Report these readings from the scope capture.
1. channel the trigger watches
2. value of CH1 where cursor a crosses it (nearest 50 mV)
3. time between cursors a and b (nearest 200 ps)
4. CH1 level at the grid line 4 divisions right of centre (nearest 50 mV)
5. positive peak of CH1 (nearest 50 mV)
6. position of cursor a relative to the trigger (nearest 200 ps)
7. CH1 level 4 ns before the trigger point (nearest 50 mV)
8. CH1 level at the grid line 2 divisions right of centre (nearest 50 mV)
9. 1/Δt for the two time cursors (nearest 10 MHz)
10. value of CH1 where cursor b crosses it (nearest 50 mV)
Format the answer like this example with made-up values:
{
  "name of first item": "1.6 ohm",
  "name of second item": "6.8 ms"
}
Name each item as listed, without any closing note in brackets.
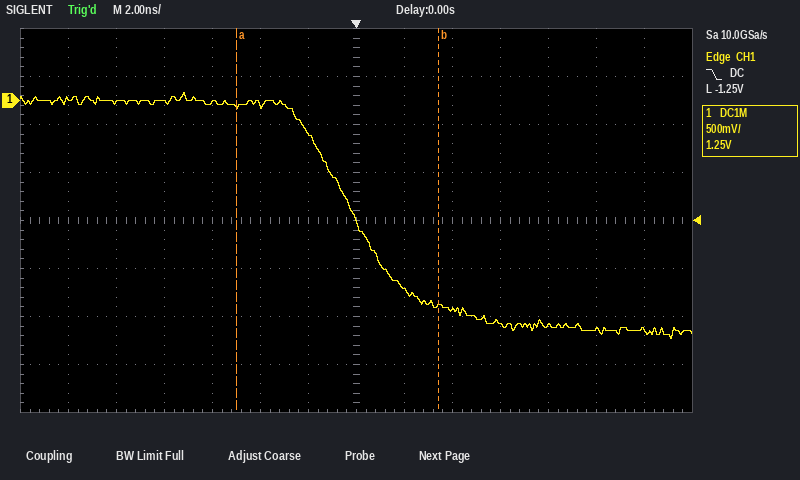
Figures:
{
  "channel the trigger watches": "CH1",
  "value of CH1 where cursor a crosses it": "-50 mV",
  "time between cursors a and b": "8.4 ns",
  "CH1 level at the grid line 4 divisions right of centre": "-2.35 V",
  "positive peak of CH1": "100 mV",
  "position of cursor a relative to the trigger": "-5.0 ns",
  "CH1 level 4 ns before the trigger point": "-50 mV",
  "CH1 level at the grid line 2 divisions right of centre": "-2.20 V",
  "1/Δt for the two time cursors": "120 MHz",
  "value of CH1 where cursor b crosses it": "-2.15 V"
}
